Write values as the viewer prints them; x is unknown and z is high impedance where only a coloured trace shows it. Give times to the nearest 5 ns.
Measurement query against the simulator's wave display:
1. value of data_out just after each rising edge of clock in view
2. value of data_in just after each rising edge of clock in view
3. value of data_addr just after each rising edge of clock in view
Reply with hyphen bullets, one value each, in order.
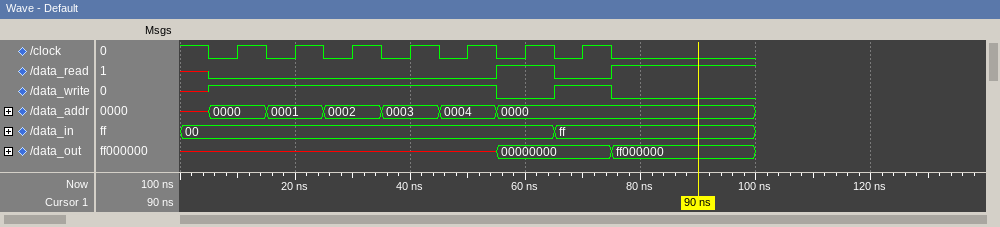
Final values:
- x, x, x, x, x, 00000000, 00000000
- 00, 00, 00, 00, 00, 00, ff
- 0000, 0001, 0002, 0003, 0004, 0000, 0000
